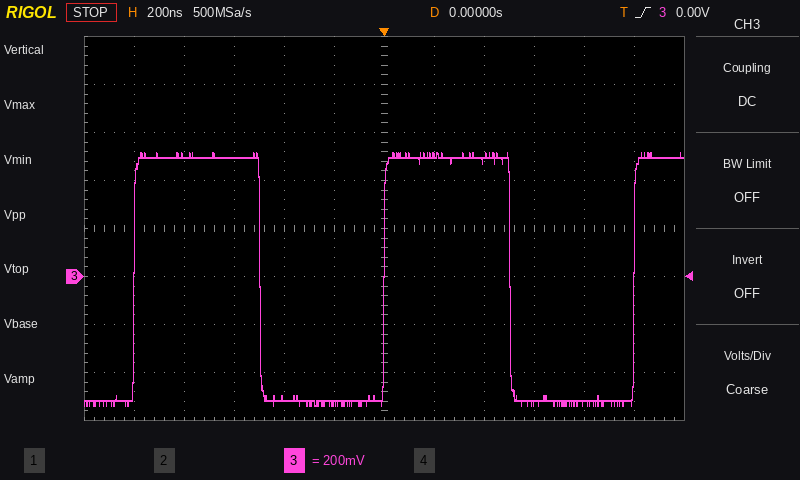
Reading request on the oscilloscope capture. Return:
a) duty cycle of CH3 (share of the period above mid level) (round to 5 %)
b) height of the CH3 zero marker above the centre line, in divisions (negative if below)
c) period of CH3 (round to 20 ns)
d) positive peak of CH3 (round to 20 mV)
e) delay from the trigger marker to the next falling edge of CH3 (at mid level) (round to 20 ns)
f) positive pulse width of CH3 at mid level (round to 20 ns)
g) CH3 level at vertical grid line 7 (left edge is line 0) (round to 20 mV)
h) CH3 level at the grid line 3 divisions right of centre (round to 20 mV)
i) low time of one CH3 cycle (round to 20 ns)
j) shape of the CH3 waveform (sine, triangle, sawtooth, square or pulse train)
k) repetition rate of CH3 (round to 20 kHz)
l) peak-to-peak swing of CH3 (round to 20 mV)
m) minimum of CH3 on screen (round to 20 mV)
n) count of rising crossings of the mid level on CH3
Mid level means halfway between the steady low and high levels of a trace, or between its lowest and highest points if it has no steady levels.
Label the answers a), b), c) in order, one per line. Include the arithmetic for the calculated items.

a) 500 ns / 1.00 µs ≈ 50 %
b) -1.0 div
c) 1.00 µs
d) 520 mV
e) 500 ns
f) 500 ns
g) 500 mV
h) -520 mV
i) 500 ns
j) square
k) 1 / 1.00 µs ≈ 1.00 MHz
l) 520 mV − (-540 mV) = 1.06 V
m) -540 mV
n) 3
